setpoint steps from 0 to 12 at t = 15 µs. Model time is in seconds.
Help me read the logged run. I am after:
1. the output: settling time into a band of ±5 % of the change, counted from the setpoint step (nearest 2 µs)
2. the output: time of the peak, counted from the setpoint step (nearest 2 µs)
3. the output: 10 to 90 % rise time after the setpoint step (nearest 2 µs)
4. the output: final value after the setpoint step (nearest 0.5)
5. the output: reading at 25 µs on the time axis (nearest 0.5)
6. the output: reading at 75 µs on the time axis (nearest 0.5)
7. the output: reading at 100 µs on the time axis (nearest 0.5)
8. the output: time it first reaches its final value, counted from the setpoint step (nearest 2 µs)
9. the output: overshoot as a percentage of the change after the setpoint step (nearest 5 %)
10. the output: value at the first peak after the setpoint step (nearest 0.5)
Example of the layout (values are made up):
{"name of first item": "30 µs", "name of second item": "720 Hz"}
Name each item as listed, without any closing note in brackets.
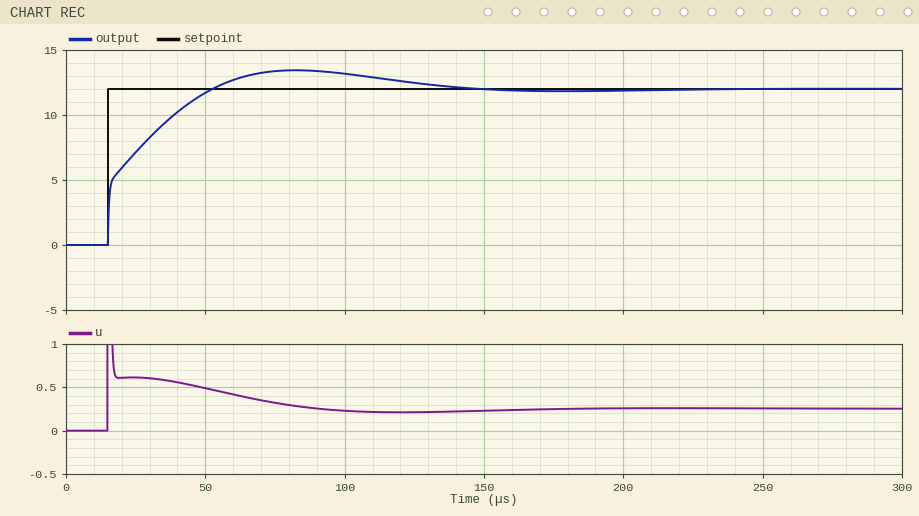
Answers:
{"the output: settling time into a band of ±5 % of the change, counted from the setpoint step": "106 µs", "the output: time of the peak, counted from the setpoint step": "68 µs", "the output: 10 to 90 % rise time after the setpoint step": "28 µs", "the output: final value after the setpoint step": "12.0", "the output: reading at 25 µs on the time axis": "7.0", "the output: reading at 75 µs on the time axis": "13.5", "the output: reading at 100 µs on the time axis": "13.0", "the output: time it first reaches its final value, counted from the setpoint step": "38 µs", "the output: overshoot as a percentage of the change after the setpoint step": "10 %", "the output: value at the first peak after the setpoint step": "13.5"}
